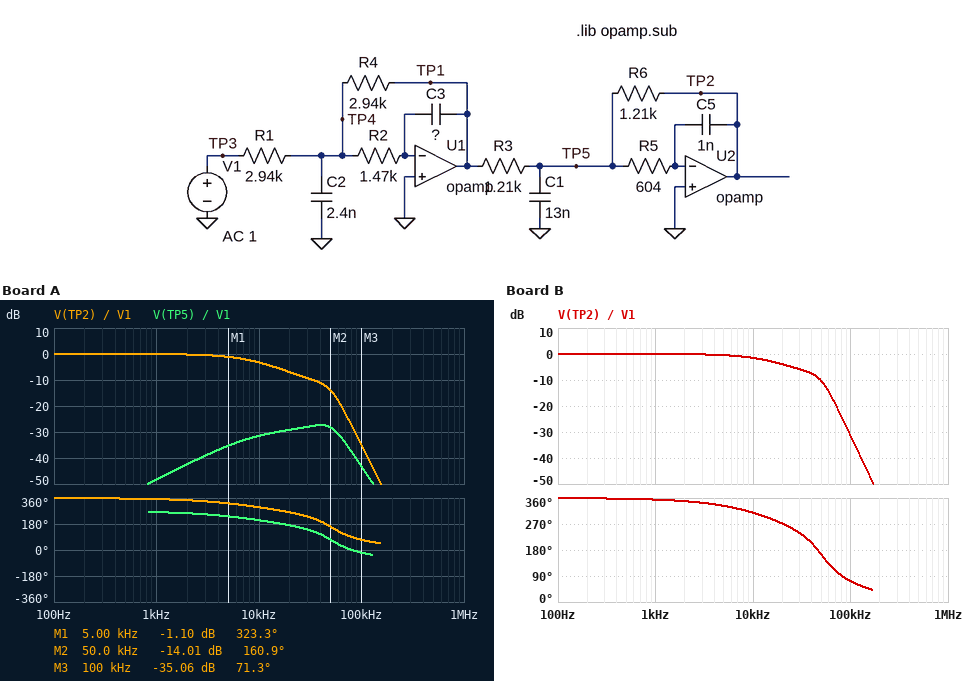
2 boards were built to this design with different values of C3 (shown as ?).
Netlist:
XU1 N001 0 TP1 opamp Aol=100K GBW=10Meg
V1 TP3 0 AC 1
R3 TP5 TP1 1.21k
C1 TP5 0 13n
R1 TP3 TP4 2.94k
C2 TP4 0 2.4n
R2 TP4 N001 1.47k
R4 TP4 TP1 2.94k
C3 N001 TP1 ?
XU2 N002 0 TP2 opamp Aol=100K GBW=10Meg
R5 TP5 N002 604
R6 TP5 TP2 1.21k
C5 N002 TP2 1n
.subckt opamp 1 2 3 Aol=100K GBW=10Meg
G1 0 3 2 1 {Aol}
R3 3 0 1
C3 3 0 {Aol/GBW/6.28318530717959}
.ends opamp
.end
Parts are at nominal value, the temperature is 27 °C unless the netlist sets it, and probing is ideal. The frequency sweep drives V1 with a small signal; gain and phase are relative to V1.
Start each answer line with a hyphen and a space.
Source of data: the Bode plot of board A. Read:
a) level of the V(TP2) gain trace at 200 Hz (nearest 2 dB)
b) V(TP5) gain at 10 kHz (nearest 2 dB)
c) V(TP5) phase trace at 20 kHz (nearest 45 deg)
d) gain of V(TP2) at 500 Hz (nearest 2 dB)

- 0 dB
- -32 dB
- 180 deg
- 0 dB
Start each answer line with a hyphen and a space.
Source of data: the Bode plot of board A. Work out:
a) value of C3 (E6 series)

- 3.3 nF
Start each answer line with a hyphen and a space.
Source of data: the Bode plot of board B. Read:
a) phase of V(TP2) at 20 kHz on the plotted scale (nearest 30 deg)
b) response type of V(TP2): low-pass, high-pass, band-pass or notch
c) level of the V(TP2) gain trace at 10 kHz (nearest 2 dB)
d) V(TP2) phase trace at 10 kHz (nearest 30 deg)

- 270 deg
- low-pass
- -2 dB
- 300 deg
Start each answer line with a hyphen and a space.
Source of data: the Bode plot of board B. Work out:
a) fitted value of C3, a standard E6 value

- 2.2 nF
